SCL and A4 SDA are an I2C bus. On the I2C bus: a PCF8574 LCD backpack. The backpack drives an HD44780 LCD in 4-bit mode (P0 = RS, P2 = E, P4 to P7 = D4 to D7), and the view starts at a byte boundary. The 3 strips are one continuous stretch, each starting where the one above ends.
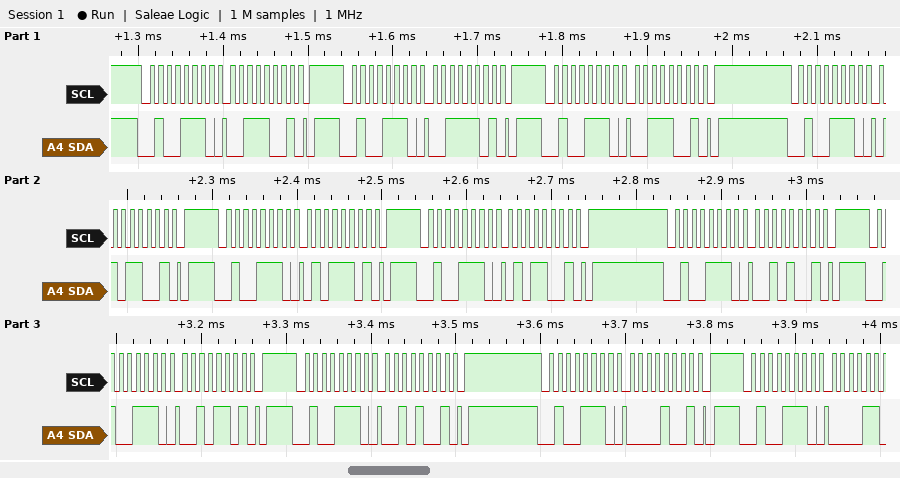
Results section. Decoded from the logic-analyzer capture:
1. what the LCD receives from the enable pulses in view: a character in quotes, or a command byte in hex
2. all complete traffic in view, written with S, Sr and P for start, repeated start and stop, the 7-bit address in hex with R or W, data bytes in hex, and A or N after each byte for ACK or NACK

'5'
S 27W A 39 A P S 27W A 3D A P S 27W A 39 A P S 27W A 59 A P S 27W A 5D A P S 27W A 59 A P S 27W A 29 A P S 27W A 2D A P S 27W A 29 A P S 27W A 09 A P S 27W A
